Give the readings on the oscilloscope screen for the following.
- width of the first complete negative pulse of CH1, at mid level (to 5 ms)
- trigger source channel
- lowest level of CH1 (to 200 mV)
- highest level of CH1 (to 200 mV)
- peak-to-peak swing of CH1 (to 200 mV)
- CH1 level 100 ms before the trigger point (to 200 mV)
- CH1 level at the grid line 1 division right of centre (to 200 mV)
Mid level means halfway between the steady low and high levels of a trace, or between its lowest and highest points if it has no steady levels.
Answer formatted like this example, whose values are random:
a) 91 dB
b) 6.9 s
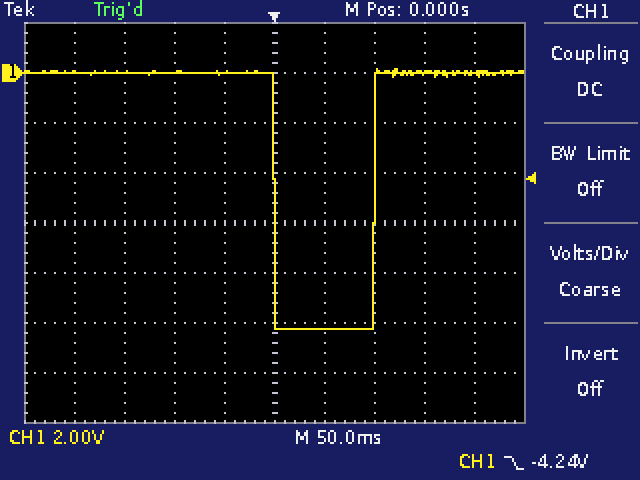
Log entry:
a) 100 ms
b) CH1
c) -10.2 V
d) 200 mV
e) 10.4 V
f) 0.0 V
g) -10.2 V
